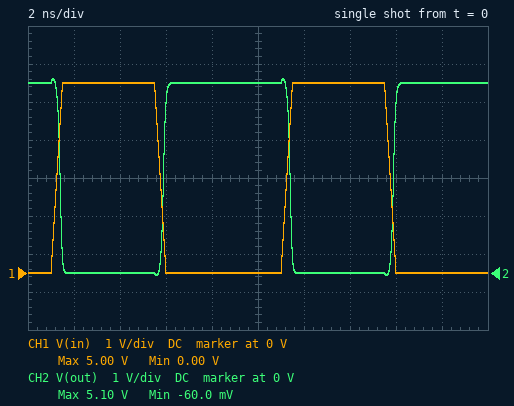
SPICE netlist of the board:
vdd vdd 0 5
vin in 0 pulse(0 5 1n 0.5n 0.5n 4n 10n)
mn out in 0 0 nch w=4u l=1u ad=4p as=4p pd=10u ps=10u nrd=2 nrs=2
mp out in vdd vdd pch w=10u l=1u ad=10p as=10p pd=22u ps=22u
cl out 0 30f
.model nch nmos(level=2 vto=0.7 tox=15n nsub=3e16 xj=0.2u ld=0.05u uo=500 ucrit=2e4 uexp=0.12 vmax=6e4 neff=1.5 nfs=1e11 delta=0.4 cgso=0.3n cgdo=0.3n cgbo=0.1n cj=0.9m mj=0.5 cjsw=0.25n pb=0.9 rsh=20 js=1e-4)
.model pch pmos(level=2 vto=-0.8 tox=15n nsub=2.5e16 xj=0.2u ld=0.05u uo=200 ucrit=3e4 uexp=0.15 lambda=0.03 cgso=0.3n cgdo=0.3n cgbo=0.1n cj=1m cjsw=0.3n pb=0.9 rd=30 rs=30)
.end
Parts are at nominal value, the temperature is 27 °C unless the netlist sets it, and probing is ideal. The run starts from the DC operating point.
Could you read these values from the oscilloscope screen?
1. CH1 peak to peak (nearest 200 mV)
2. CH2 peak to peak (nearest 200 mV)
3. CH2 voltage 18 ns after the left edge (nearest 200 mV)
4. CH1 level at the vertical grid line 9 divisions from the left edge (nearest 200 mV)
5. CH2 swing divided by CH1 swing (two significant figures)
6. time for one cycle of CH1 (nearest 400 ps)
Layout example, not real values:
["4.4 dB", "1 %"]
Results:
["5.0 V", "5.2 V", "5.0 V", "0 V", "1.0", "10.0 ns"]
